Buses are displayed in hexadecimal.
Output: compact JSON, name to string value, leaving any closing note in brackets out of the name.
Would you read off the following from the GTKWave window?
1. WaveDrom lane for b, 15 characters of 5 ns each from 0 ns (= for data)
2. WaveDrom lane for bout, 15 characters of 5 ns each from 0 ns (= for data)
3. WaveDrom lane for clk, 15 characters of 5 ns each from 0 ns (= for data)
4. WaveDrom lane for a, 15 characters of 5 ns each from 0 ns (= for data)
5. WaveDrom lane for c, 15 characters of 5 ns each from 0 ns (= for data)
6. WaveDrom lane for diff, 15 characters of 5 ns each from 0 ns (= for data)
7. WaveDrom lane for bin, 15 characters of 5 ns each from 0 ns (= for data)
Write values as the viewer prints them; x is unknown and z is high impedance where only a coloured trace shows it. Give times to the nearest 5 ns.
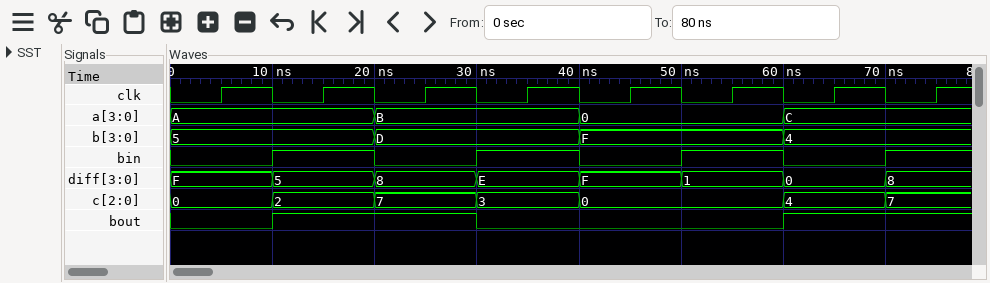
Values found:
{"WaveDrom lane for b, 15 characters of 5 ns each from 0 ns": "{name: 'b', wave: '=...=...=...=..', data: '5 D F 4'}", "WaveDrom lane for bout, 15 characters of 5 ns each from 0 ns": "{name: 'bout', wave: '0.1...0.....1..'}", "WaveDrom lane for clk, 15 characters of 5 ns each from 0 ns": "{name: 'clk', wave: '010101010101010'}", "WaveDrom lane for a, 15 characters of 5 ns each from 0 ns": "{name: 'a', wave: '=...=...=...=..', data: 'A B 0 C'}", "WaveDrom lane for c, 15 characters of 5 ns each from 0 ns": "{name: 'c', wave: '=.=.=.=.=...=.=', data: '0 2 7 3 0 4 7'}", "WaveDrom lane for diff, 15 characters of 5 ns each from 0 ns": "{name: 'diff', wave: '=.=.=.=.=.=.=.=', data: 'F 5 8 E F 1 0 8'}", "WaveDrom lane for bin, 15 characters of 5 ns each from 0 ns": "{name: 'bin', wave: '0.1.0.1.0.1.0.1'}"}
